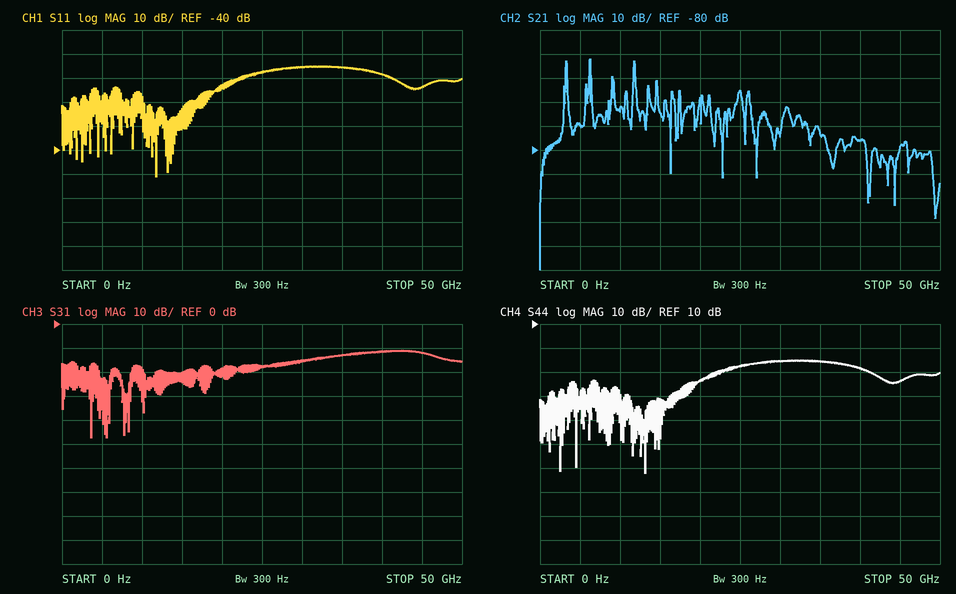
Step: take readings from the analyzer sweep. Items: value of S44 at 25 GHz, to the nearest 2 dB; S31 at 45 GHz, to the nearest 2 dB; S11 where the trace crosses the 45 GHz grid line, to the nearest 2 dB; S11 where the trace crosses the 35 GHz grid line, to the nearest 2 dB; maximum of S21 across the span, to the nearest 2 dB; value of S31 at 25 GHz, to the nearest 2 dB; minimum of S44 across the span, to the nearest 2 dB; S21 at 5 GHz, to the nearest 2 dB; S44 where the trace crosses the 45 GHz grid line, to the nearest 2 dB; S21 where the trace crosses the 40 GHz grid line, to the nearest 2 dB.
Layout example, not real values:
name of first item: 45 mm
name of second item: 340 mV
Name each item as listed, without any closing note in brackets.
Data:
value of S44 at 25 GHz, to the nearest 2 dB: -8 dB
S31 at 45 GHz, to the nearest 2 dB: -12 dB
S11 where the trace crosses the 45 GHz grid line, to the nearest 2 dB: -14 dB
S11 where the trace crosses the 35 GHz grid line, to the nearest 2 dB: -6 dB
maximum of S21 across the span, to the nearest 2 dB: -42 dB
value of S31 at 25 GHz, to the nearest 2 dB: -18 dB
minimum of S44 across the span, to the nearest 2 dB: -52 dB
S21 at 5 GHz, to the nearest 2 dB: -70 dB
S44 where the trace crosses the 45 GHz grid line, to the nearest 2 dB: -14 dB
S21 where the trace crosses the 40 GHz grid line, to the nearest 2 dB: -76 dB
